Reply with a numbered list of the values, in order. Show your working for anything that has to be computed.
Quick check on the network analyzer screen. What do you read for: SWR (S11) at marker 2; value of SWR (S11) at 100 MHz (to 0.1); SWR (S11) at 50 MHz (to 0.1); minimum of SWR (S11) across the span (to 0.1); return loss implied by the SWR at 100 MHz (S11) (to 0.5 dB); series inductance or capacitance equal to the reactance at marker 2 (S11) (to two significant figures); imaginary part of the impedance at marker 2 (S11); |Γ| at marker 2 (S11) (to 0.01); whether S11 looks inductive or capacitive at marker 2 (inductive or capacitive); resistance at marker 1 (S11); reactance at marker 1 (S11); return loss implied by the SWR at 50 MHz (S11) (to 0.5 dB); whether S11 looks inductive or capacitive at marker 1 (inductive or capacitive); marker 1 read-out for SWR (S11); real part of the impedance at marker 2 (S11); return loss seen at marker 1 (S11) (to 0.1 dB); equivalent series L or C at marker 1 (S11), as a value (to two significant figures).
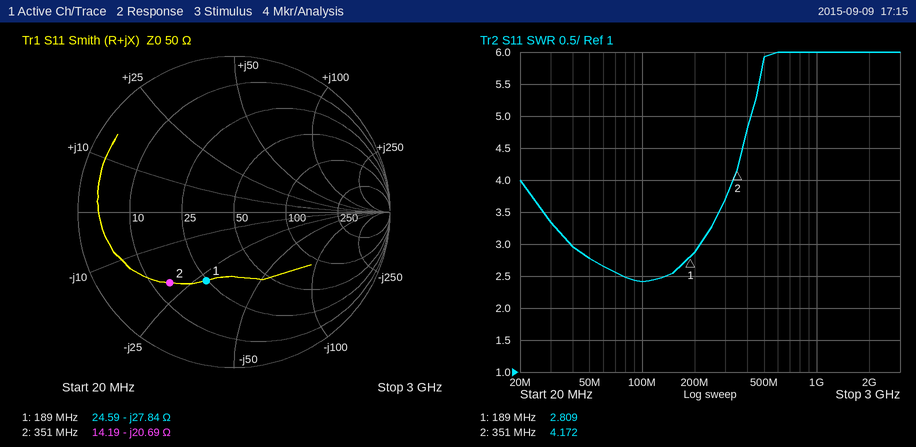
1. 4.172
2. 2.4
3. 2.8
4. 2.4
5. −20 log10((2.4 − 1)/(2.4 + 1)) ≈ 7.71 dB, so 7.5 dB to the nearest 0.5 dB
6. C = 1/(2π × 351 MHz × 20.69 Ω) ≈ 22 pF
7. -20.69 Ω
8. 0.61
9. capacitive
10. 24.59 Ω
11. -27.84 Ω
12. −20 log10((2.8 − 1)/(2.8 + 1)) ≈ 6.5 dB
13. capacitive
14. 2.809
15. 14.19 Ω
16. 6.5 dB
17. C = 1/(2π × 189 MHz × 27.84 Ω) ≈ 30 pF
